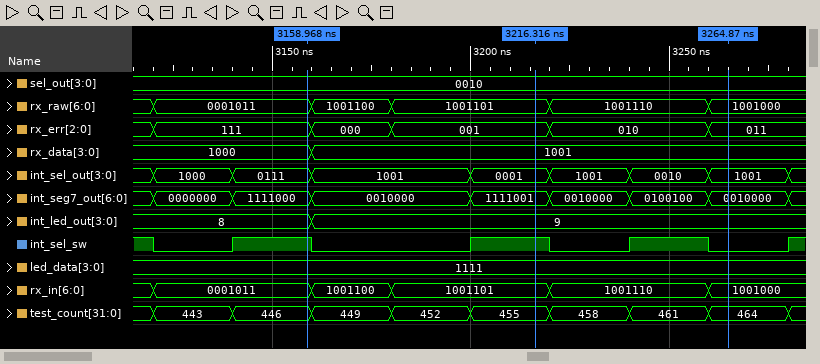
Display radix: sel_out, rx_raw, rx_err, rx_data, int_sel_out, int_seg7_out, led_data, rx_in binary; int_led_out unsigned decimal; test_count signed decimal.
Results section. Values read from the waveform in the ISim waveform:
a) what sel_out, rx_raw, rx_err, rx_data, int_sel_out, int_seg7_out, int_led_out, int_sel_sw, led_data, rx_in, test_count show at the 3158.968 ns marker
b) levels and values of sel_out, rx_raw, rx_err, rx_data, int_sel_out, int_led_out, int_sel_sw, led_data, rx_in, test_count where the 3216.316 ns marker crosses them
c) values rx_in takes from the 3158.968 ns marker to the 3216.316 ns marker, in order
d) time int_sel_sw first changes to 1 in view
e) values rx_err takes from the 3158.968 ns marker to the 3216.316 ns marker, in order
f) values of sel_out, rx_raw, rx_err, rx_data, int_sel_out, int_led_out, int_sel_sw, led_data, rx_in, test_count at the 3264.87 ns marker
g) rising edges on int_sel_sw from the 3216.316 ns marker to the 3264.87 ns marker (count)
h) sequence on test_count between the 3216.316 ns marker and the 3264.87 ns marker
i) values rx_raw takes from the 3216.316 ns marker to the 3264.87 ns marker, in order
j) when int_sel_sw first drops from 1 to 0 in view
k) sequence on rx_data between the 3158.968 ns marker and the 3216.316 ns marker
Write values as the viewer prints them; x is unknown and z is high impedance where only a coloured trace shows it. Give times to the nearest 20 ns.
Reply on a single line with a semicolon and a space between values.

sel_out=0010, rx_raw=0001011, rx_err=111, rx_data=1000, int_sel_out=0111, int_seg7_out=1111000, int_led_out=8, int_sel_sw=1, led_data=1111, rx_in=0001011, test_count=446; sel_out=0010, rx_raw=1001101, rx_err=001, rx_data=1001, int_sel_out=0001, int_led_out=9, int_sel_sw=1, led_data=1111, rx_in=1001101, test_count=455; 0001011, 1001100, 1001101; 3140 ns; 111, 000, 001; sel_out=0010, rx_raw=1001000, rx_err=011, rx_data=1001, int_sel_out=1001, int_led_out=9, int_sel_sw=0, led_data=1111, rx_in=1001000, test_count=464; 1; 455, 458, 461, 464; 1001101, 1001110, 1001000; 3120 ns; 1000, 1001
